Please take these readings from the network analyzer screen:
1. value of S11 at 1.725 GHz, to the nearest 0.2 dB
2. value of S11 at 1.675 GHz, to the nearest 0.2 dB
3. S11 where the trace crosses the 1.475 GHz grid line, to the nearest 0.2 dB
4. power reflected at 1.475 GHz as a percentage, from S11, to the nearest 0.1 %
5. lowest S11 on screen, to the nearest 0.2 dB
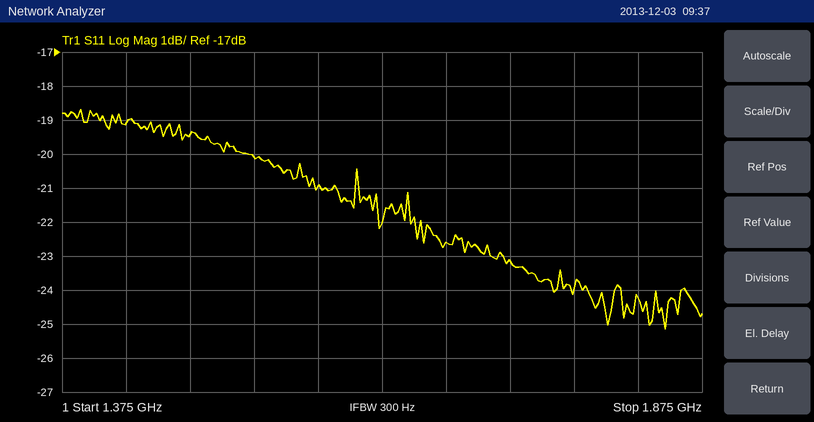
-23.2 dB
-22.6 dB
-19.4 dB
1.1 %
-25.2 dB
